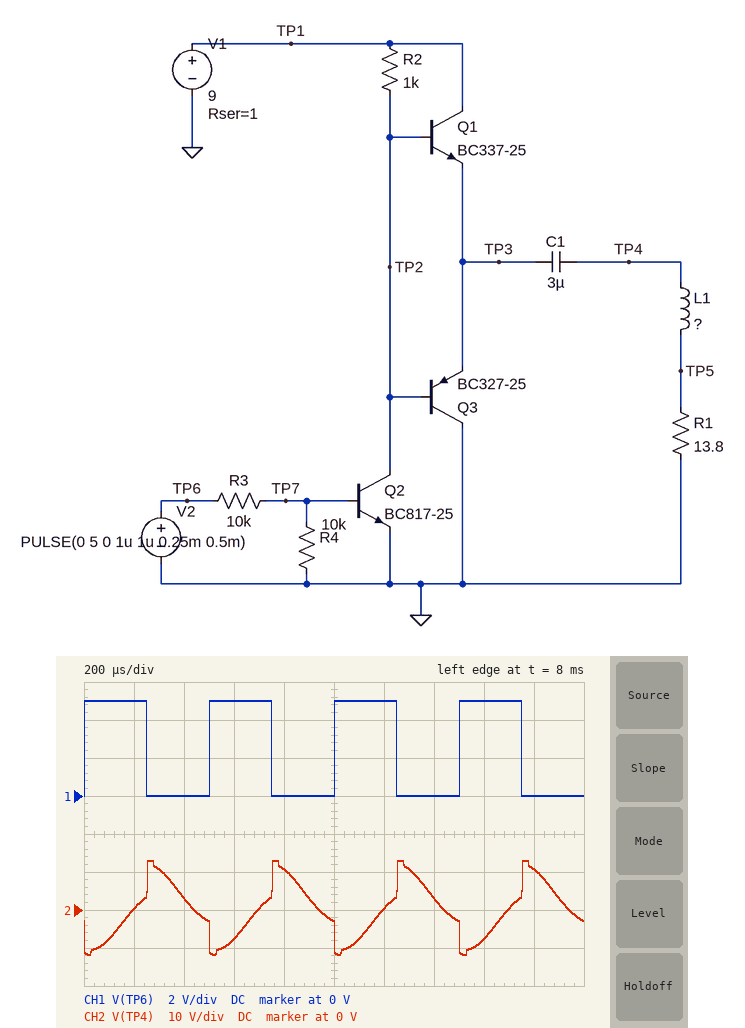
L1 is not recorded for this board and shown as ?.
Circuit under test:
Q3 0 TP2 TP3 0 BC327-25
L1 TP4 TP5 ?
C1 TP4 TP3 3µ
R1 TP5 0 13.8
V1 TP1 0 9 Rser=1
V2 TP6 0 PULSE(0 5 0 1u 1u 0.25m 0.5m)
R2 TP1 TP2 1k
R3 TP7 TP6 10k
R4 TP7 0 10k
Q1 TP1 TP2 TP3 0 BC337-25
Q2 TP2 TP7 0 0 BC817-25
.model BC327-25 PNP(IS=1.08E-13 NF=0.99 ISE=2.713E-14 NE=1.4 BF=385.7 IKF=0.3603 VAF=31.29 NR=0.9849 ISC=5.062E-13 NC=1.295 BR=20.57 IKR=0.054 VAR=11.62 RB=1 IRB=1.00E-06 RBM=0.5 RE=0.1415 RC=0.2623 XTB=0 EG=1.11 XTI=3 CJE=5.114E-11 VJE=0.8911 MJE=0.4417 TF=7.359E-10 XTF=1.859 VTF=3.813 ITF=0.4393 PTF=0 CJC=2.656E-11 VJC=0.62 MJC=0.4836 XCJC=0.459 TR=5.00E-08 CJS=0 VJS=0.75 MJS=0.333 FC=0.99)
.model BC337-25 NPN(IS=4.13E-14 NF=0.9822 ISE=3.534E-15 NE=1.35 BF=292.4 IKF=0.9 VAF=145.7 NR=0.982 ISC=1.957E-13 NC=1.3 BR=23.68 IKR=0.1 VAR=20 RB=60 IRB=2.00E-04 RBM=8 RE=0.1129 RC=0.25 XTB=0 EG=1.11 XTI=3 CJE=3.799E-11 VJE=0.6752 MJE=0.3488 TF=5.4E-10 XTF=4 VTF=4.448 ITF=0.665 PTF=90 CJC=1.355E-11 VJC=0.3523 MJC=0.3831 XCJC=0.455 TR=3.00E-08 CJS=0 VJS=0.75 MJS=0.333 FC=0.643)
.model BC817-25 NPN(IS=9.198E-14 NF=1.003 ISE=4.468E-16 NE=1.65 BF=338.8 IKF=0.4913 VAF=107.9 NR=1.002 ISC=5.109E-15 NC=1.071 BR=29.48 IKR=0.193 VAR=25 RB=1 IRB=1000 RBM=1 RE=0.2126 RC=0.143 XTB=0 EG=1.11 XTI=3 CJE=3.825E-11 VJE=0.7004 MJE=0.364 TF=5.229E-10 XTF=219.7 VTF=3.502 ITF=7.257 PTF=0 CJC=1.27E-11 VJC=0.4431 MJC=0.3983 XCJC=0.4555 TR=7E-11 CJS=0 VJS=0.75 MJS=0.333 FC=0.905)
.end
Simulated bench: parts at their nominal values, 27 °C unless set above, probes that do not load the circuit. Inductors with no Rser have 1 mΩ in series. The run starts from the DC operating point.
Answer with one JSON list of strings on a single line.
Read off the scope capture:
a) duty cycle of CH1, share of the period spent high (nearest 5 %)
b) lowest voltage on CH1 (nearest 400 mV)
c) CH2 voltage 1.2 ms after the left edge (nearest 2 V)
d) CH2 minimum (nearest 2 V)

["50 %", "0 V", "0 V", "-12 V"]
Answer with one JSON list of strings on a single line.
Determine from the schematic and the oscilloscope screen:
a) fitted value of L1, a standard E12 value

["2.7 mH"]
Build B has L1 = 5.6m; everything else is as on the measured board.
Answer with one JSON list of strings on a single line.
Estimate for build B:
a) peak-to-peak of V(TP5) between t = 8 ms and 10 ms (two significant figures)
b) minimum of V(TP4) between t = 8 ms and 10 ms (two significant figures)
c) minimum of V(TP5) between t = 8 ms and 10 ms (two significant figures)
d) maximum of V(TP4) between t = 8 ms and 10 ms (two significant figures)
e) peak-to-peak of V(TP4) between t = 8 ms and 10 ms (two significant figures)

["3.3 V", "-7.9 V", "-1.7 V", "8.3 V", "16 V"]
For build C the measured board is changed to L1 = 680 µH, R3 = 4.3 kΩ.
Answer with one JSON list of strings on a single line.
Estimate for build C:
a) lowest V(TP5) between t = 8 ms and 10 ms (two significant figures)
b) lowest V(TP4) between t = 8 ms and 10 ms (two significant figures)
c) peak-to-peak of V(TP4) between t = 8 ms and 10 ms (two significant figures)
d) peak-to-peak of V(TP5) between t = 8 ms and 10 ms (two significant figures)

["-4.2 V", "-8.3 V", "17 V", "8.1 V"]
